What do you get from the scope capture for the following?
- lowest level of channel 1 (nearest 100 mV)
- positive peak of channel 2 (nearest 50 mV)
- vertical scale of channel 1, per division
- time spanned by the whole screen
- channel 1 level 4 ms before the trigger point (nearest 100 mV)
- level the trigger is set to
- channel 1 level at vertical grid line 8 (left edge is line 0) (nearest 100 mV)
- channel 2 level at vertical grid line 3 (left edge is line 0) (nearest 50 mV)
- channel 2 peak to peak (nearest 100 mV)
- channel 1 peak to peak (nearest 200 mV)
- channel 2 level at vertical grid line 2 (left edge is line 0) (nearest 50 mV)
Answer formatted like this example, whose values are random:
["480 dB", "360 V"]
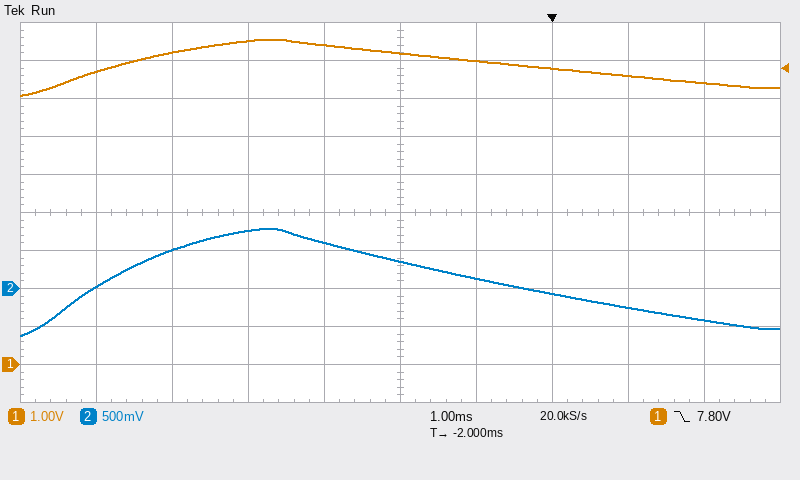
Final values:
["7.1 V", "800 mV", "1 V", "10 ms", "8.5 V", "7.80 V", "7.6 V", "750 mV", "1.40 V", "1.4 V", "500 mV"]
